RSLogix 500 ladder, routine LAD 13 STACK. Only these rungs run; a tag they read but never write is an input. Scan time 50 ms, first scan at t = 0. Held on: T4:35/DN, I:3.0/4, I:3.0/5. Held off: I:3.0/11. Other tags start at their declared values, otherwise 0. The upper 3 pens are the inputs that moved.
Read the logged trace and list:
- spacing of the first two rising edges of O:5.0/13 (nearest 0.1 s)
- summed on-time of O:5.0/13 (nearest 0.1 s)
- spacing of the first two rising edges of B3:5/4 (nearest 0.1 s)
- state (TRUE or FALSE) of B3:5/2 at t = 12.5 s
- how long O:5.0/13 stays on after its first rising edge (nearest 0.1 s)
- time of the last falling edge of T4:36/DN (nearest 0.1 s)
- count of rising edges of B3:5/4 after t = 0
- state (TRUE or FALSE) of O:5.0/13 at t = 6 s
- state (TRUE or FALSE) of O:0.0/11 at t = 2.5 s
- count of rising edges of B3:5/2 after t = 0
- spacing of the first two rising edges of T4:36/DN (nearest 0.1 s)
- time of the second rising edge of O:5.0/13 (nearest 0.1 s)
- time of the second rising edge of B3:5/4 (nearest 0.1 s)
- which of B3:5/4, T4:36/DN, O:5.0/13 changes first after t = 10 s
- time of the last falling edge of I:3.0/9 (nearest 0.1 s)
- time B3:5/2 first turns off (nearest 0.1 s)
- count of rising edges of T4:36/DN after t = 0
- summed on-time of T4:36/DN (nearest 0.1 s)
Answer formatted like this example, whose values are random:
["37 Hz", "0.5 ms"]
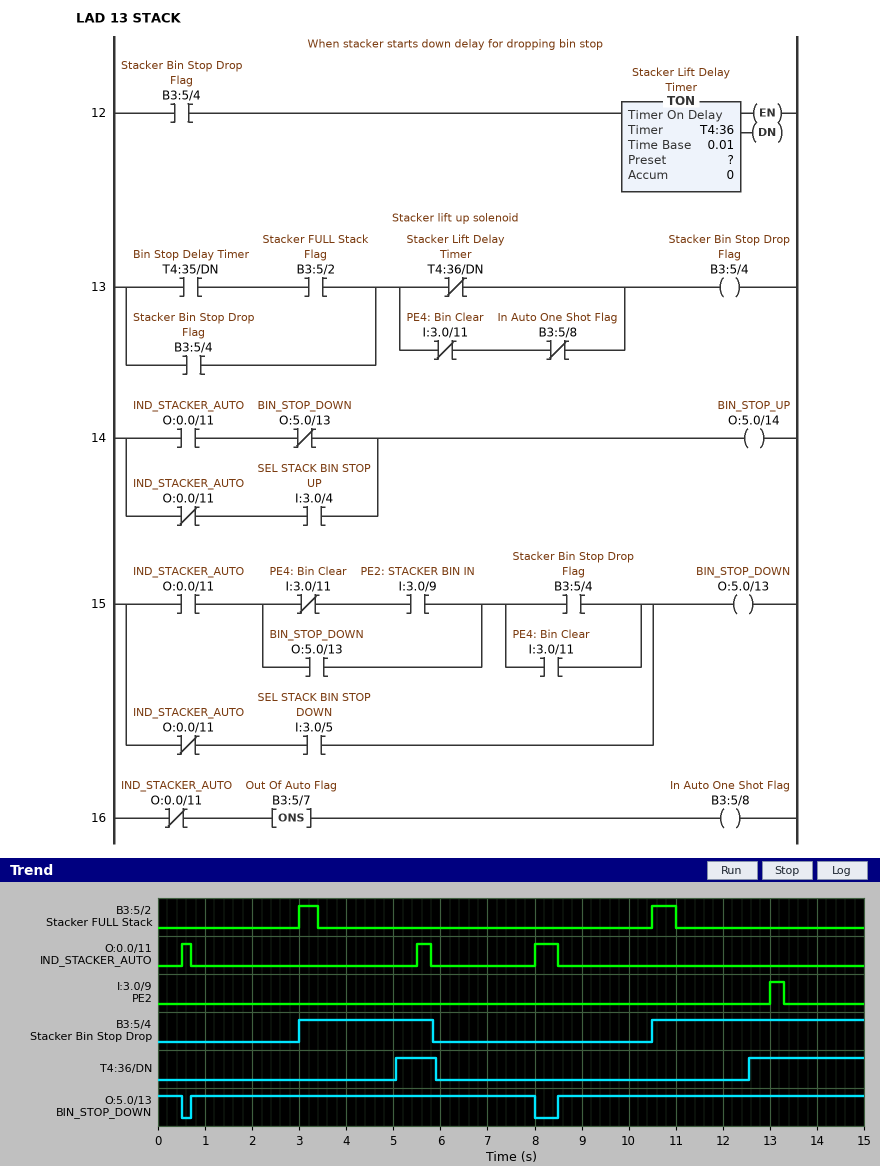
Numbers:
["7.8 s", "14.3 s", "7.5 s", "FALSE", "7.3 s", "5.9 s", "2", "TRUE", "FALSE", "2", "7.5 s", "8.5 s", "10.5 s", "B3:5/4", "13.3 s", "3.4 s", "2", "3.3 s"]
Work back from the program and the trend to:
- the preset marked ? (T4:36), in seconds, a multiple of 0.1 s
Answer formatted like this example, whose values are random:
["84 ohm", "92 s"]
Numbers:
["2.0 s"]
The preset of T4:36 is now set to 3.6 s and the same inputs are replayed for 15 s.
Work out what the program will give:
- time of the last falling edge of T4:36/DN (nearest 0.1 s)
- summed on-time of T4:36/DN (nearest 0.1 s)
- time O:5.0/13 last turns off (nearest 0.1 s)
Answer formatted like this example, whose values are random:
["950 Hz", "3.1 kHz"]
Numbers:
["8.6 s", "2.8 s", "0.5 s"]
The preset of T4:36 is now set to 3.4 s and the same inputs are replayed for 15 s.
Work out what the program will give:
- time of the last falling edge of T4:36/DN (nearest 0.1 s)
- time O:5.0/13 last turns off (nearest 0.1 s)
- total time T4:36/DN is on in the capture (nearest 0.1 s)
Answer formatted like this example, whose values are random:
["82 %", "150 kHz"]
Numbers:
["8.6 s", "0.5 s", "3.2 s"]
